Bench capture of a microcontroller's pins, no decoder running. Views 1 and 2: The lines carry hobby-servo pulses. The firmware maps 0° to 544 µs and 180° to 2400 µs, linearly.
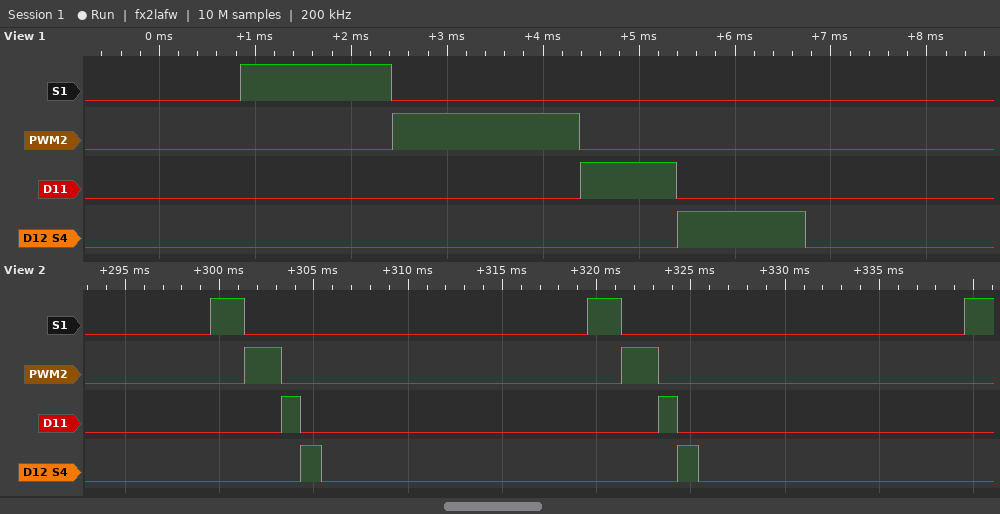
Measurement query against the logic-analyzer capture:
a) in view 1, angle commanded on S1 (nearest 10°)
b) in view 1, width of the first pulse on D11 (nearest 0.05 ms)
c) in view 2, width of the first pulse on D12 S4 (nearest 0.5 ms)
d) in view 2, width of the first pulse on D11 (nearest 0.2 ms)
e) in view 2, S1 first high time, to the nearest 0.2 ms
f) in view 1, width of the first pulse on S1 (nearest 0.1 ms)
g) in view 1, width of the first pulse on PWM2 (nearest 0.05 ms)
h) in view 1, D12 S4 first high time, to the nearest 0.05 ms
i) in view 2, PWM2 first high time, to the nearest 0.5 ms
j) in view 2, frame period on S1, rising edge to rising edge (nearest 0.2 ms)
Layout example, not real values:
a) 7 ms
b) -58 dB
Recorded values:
a) 100°
b) 1.00 ms
c) 1.0 ms
d) 1.0 ms
e) 1.8 ms
f) 1.6 ms
g) 1.95 ms
h) 1.35 ms
i) 2.0 ms
j) 20.0 ms
